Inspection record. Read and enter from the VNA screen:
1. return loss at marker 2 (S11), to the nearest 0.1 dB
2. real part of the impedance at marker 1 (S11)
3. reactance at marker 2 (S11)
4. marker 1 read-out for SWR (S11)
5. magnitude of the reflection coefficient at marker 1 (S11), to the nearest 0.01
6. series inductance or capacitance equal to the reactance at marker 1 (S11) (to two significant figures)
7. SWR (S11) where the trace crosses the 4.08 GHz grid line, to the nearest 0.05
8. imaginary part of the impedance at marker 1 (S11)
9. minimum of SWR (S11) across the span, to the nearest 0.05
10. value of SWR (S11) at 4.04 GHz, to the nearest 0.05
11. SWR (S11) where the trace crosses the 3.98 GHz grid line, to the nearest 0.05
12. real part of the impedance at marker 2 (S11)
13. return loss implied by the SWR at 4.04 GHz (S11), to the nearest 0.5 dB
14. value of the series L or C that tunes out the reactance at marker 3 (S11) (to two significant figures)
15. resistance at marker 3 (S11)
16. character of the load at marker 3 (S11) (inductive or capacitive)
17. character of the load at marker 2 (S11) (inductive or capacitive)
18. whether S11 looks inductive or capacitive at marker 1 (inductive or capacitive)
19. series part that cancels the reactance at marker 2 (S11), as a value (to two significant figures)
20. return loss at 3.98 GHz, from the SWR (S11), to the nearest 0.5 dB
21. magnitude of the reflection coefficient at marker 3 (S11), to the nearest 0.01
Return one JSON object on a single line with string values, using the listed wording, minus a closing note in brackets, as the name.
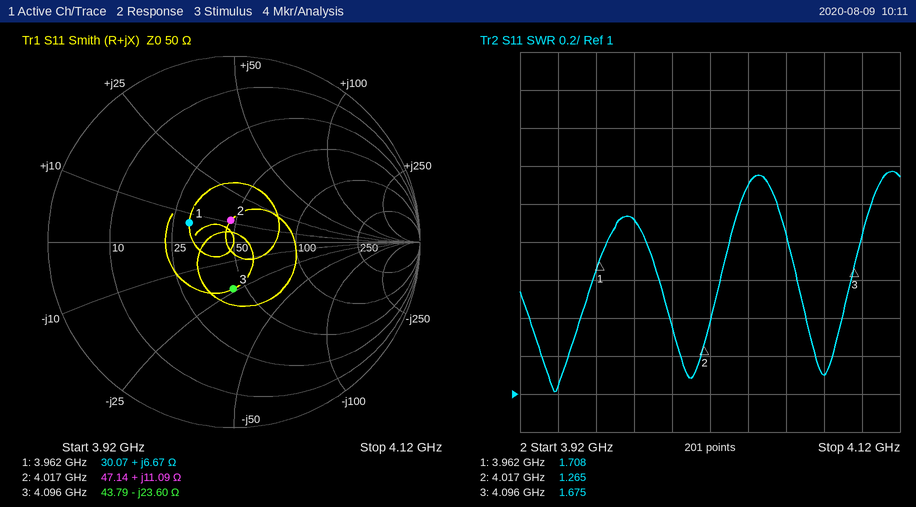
{"return loss at marker 2 (S11), to the nearest 0.1 dB": "18.6 dB", "real part of the impedance at marker 1": "30.07 Ω", "reactance at marker 2": "+11.09 Ω", "marker 1 read-out for SWR": "1.708", "magnitude of the reflection coefficient at marker 1 (S11), to the nearest 0.01": "0.26", "series inductance or capacitance equal to the reactance at marker 1 (S11)": "270 pH", "SWR (S11) where the trace crosses the 4.08 GHz grid line, to the nearest 0.05": "1.10", "imaginary part of the impedance at marker 1": "+6.67 Ω", "minimum of SWR (S11) across the span, to the nearest 0.05": "1.00", "value of SWR (S11) at 4.04 GHz, to the nearest 0.05": "2.10", "SWR (S11) where the trace crosses the 3.98 GHz grid line, to the nearest 0.05": "1.90", "real part of the impedance at marker 2": "47.14 Ω", "return loss implied by the SWR at 4.04 GHz (S11), to the nearest 0.5 dB": "9.0 dB", "value of the series L or C that tunes out the reactance at marker 3 (S11)": "920 pH", "resistance at marker 3": "43.79 Ω", "character of the load at marker 3 (S11)": "capacitive", "character of the load at marker 2 (S11)": "inductive", "whether S11 looks inductive or capacitive at marker 1": "inductive", "series part that cancels the reactance at marker 2 (S11), as a value": "3.6 pF", "return loss at 3.98 GHz, from the SWR (S11), to the nearest 0.5 dB": "10.0 dB", "magnitude of the reflection coefficient at marker 3 (S11), to the nearest 0.01": "0.25"}
